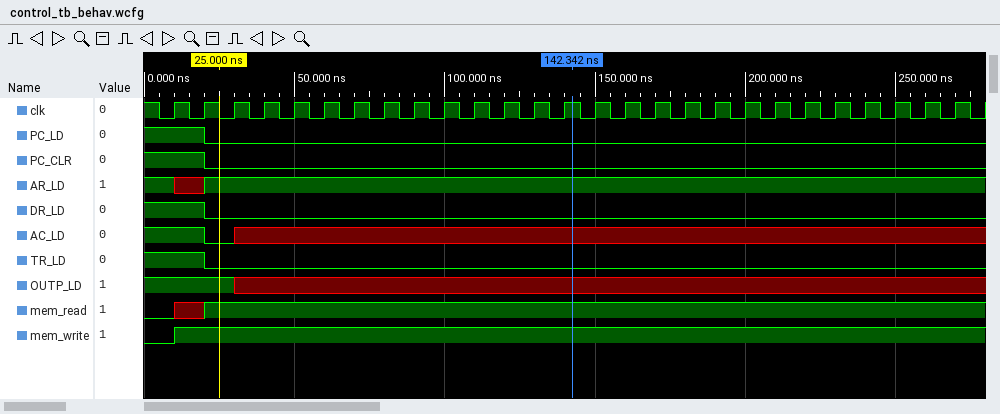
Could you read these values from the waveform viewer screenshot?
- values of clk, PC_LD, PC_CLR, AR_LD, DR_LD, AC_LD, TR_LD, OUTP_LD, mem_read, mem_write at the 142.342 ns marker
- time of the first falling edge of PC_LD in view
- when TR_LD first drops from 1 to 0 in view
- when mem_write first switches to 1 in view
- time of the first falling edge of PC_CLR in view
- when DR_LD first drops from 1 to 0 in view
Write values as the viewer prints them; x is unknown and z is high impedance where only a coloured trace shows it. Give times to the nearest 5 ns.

clk=1, PC_LD=0, PC_CLR=0, AR_LD=1, DR_LD=0, AC_LD=x, TR_LD=0, OUTP_LD=x, mem_read=1, mem_write=1
20 ns
20 ns
10 ns
20 ns
20 ns
